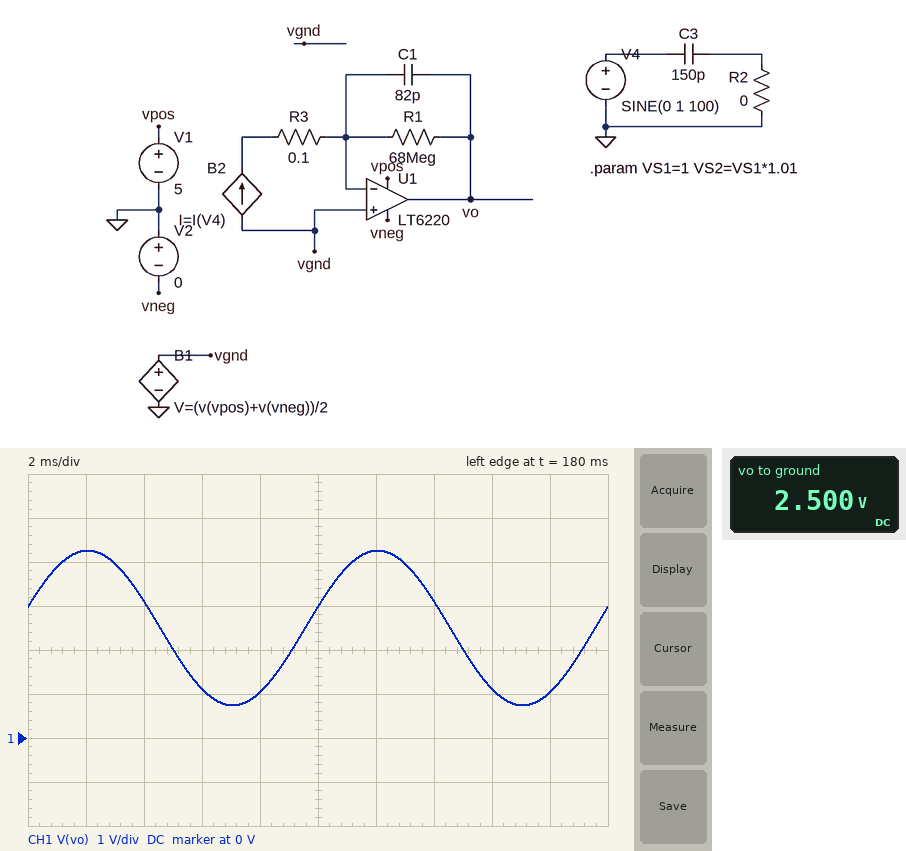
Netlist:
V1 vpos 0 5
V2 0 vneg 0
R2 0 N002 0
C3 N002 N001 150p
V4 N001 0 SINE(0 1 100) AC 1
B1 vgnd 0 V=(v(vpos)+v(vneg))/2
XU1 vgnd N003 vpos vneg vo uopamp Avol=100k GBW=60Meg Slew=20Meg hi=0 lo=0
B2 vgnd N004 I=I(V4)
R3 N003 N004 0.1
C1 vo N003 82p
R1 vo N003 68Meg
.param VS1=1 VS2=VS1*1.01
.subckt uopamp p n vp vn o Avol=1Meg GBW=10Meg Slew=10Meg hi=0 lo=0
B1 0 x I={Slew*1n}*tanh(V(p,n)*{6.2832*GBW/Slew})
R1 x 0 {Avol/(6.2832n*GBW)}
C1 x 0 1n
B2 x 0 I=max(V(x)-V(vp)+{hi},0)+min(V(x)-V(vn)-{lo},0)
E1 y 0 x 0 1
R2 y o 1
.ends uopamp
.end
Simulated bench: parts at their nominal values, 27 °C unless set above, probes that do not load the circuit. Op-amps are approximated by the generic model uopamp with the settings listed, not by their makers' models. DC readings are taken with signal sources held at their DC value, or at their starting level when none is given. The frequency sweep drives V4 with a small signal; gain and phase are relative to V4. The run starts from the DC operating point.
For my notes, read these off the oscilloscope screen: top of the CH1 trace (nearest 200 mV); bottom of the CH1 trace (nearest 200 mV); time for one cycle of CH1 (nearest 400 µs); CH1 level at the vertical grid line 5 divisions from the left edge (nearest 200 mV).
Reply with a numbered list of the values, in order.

1. 4.2 V
2. 800 mV
3. 10.0 ms
4. 3.0 V
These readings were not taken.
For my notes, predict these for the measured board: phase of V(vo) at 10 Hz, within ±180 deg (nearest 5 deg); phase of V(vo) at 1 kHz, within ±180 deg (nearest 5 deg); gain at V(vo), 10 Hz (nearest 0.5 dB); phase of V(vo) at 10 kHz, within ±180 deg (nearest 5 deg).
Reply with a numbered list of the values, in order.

1. 70 deg
2. 0 deg
3. -4.5 dB
4. 0 deg
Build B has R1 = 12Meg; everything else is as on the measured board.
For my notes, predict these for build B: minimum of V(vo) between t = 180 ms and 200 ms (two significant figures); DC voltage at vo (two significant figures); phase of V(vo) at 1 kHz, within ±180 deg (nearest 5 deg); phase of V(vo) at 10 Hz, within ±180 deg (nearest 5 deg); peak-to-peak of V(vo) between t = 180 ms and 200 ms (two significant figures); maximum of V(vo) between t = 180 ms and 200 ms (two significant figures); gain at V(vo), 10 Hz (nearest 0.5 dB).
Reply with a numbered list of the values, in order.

1. 1.5 V
2. 2.5 V
3. 10 deg
4. 85 deg
5. 1.9 V
6. 3.5 V
7. -19.0 dB
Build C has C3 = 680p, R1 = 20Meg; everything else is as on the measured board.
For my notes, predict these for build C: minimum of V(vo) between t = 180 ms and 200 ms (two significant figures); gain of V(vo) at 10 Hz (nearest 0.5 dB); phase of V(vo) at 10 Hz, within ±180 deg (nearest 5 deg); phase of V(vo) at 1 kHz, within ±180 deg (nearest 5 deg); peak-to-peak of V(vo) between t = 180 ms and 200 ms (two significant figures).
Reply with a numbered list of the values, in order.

1. -20 mV
2. -1.5 dB
3. 85 deg
4. 5 deg
5. 5.0 V
